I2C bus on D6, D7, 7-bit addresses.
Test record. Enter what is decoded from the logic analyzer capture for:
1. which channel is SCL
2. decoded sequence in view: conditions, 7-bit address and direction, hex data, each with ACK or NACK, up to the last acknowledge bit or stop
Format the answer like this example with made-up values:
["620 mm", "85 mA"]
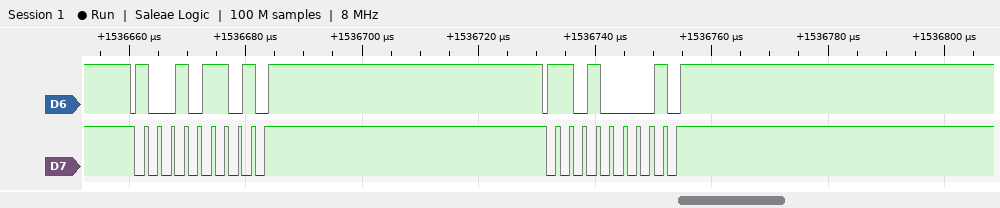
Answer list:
["D7", "start, address 4B write NACK, stop, start, address 68 write NACK, stop"]
